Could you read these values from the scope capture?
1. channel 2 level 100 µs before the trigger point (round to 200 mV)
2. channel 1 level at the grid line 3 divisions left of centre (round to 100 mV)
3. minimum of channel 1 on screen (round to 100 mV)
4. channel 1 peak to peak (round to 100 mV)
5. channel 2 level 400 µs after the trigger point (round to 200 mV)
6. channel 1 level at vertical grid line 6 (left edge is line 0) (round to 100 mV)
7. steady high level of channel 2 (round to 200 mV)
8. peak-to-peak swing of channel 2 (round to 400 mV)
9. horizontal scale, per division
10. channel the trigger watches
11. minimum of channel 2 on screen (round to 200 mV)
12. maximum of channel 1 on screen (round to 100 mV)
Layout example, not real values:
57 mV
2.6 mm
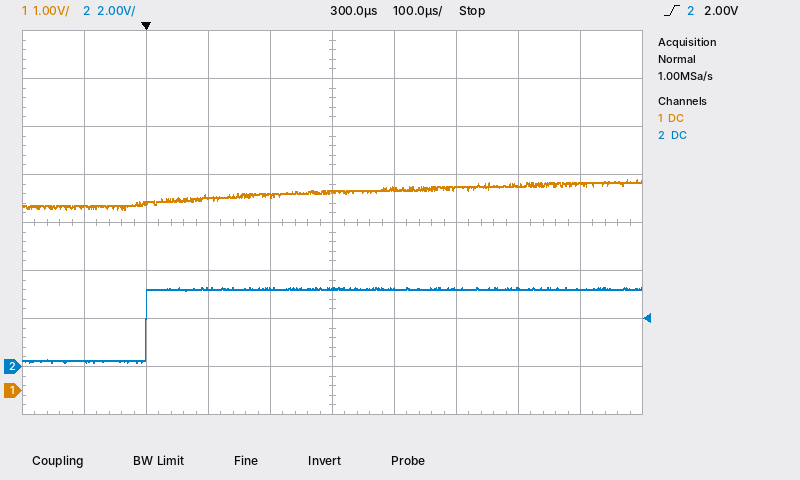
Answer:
200 mV
3.9 V
3.8 V
600 mV
3.2 V
4.2 V
3.2 V
3.2 V
100 µs
channel 2
200 mV
4.4 V
